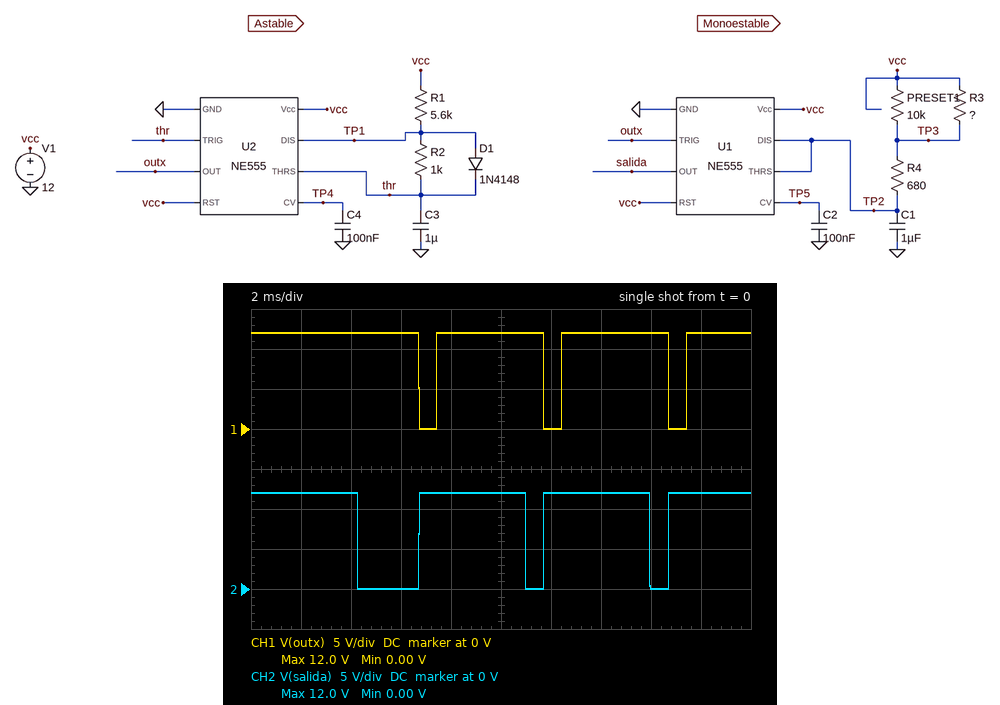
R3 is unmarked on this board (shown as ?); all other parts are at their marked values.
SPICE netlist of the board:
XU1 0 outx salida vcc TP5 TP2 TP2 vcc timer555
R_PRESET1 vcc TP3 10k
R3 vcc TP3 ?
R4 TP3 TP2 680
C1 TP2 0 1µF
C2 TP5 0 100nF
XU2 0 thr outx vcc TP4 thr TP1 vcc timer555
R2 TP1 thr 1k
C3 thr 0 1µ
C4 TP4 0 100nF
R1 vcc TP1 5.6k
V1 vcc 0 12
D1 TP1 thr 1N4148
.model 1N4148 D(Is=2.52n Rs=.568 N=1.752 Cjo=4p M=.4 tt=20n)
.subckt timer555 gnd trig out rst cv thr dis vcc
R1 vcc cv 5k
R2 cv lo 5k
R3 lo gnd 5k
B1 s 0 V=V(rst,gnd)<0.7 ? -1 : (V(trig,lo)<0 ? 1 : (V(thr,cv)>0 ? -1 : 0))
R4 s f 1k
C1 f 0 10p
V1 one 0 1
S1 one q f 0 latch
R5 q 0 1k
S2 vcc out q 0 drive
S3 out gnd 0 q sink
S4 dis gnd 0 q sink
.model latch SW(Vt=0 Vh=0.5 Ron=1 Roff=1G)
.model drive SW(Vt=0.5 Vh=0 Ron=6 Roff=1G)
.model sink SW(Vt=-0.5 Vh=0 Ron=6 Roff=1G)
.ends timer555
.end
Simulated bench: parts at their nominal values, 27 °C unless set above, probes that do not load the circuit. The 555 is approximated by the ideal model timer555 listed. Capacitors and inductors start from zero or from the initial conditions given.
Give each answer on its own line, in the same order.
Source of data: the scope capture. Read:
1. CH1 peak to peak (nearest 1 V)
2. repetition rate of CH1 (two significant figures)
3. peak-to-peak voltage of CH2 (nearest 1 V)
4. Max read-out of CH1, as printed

12 V
200 Hz
12 V
12.0 V
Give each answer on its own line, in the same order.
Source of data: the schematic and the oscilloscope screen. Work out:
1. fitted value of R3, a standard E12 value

4.7 kΩ
